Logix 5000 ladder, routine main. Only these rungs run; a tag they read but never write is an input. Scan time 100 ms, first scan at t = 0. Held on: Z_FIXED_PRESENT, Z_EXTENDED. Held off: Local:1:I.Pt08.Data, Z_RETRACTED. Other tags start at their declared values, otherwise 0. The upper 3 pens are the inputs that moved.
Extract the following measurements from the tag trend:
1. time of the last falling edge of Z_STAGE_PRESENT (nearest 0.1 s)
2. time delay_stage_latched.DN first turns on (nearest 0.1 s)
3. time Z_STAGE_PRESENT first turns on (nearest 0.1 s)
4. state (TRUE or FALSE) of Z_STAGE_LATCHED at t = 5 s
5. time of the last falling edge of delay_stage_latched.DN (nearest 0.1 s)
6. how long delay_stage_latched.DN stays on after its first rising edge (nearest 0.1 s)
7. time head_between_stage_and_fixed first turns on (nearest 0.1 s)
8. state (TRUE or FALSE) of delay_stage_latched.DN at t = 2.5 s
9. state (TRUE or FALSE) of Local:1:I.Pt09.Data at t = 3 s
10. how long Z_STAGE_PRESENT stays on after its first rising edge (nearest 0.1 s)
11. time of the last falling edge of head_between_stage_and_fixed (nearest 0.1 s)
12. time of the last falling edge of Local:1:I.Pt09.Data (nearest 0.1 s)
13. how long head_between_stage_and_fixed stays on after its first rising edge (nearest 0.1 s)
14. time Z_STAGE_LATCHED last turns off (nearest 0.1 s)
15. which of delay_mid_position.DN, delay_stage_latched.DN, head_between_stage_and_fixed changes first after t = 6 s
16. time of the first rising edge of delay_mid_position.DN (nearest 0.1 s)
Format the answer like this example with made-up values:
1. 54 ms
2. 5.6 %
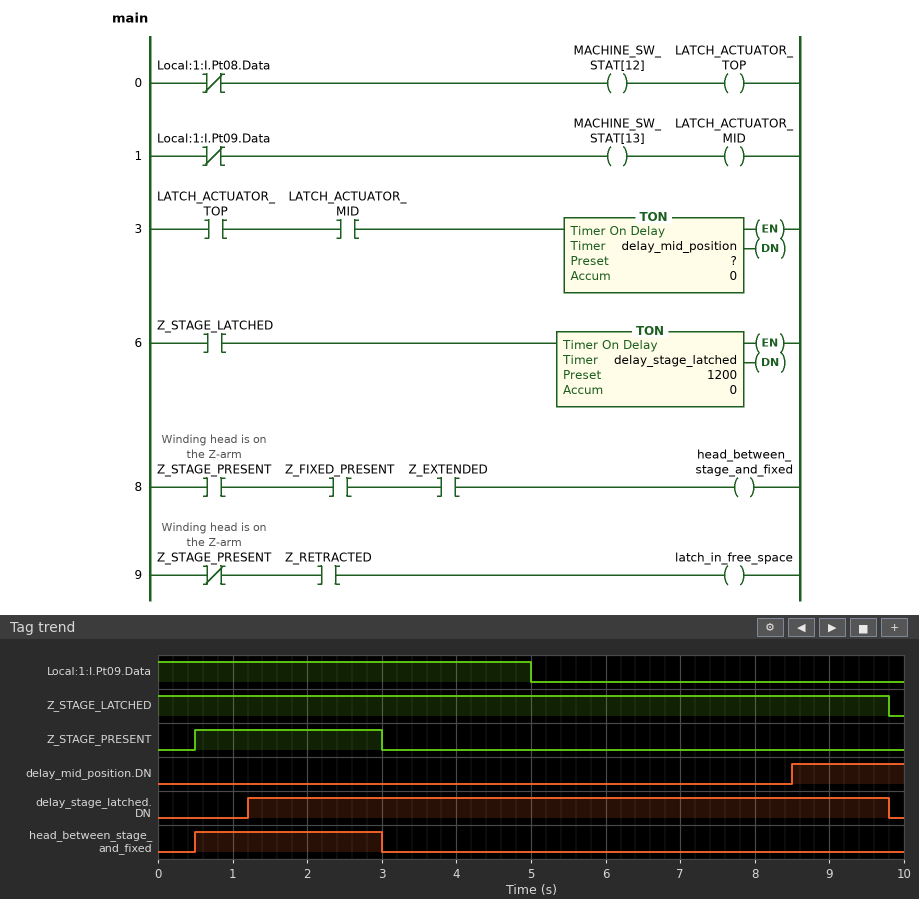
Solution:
1. 3.0 s
2. 1.2 s
3. 0.5 s
4. TRUE
5. 9.8 s
6. 8.6 s
7. 0.5 s
8. TRUE
9. TRUE
10. 2.5 s
11. 3.0 s
12. 5.0 s
13. 2.5 s
14. 9.8 s
15. delay_mid_position.DN
16. 8.5 s
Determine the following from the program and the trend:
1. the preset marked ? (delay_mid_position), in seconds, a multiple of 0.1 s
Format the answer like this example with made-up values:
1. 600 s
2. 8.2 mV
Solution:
1. 3.5 s
